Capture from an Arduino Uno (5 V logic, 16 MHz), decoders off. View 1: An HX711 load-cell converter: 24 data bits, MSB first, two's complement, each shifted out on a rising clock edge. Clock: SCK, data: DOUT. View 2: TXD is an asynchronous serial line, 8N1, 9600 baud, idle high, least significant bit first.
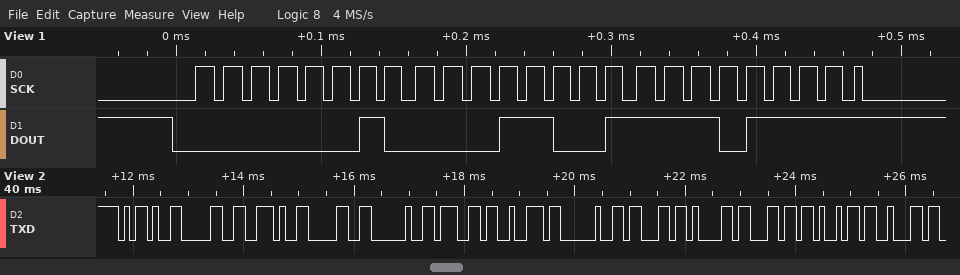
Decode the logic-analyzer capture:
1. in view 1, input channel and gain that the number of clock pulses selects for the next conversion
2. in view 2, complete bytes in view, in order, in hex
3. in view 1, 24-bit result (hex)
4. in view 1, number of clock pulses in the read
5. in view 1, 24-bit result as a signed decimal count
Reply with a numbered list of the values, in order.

1. channel A, gain 128
2. 2D 30 2E 30 20 67 72 20 63 61 6C 69 62
3. 0x0219EF
4. 25
5. 137711
